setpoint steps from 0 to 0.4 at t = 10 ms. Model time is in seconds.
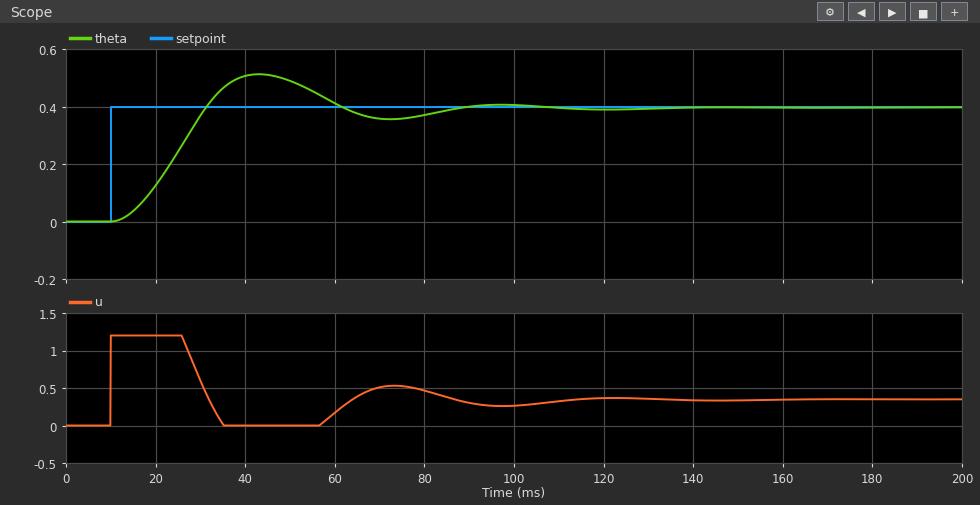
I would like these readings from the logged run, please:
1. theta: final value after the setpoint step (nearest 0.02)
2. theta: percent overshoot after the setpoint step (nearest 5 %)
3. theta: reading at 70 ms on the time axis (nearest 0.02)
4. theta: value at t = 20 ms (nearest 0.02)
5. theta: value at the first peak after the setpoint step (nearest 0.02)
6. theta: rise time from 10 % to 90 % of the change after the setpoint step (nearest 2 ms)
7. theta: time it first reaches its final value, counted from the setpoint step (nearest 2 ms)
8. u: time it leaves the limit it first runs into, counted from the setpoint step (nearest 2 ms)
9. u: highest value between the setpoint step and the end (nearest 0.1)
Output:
0.40
30 %
0.36
0.12
0.52
14 ms
22 ms
16 ms
1.2
